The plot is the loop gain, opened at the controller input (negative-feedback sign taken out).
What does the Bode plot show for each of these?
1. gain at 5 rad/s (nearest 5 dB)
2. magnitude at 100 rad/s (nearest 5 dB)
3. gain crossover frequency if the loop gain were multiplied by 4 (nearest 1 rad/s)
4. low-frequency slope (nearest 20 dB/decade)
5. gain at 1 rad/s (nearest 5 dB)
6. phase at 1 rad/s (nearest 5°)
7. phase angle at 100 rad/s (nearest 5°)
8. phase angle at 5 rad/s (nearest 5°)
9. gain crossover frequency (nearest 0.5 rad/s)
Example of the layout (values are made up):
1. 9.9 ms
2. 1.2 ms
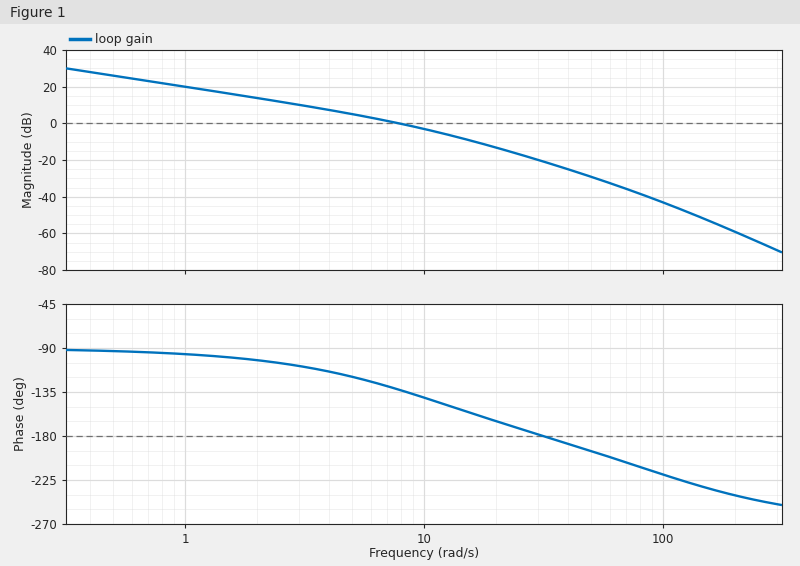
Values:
1. 5 dB
2. -45 dB
3. 19 rad/s
4. -20 dB/decade
5. 20 dB
6. -95°
7. -220°
8. -120°
9. 8.0 rad/s
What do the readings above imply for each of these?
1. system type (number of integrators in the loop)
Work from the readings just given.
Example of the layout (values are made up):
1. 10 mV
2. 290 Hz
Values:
1. 1
